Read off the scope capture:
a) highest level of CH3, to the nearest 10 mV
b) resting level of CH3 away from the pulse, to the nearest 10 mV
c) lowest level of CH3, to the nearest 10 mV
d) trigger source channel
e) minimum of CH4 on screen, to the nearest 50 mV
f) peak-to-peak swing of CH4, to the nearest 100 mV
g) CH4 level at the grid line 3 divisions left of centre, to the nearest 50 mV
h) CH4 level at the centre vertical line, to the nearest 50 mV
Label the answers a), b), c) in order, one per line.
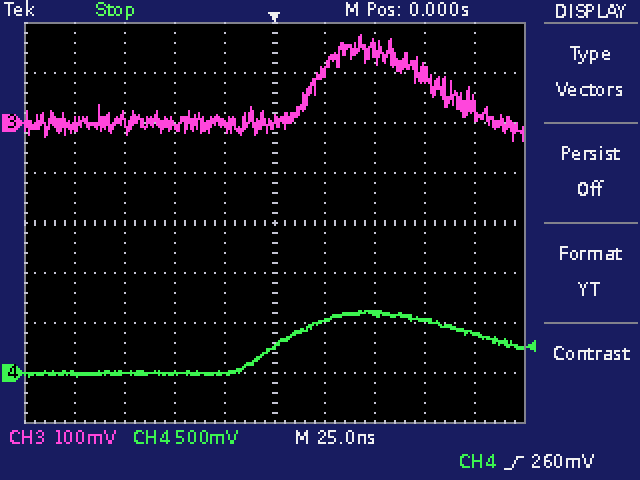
a) 180 mV
b) 0 mV
c) -40 mV
d) CH4
e) -50 mV
f) 700 mV
g) 0 mV
h) 250 mV
